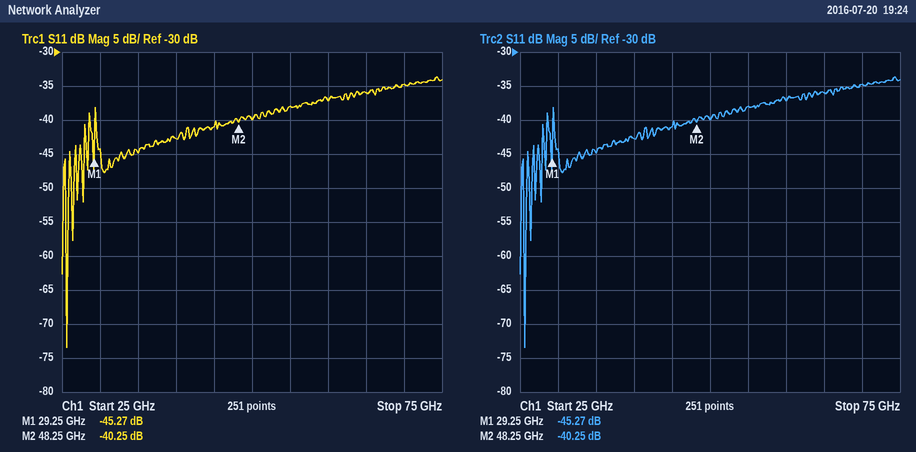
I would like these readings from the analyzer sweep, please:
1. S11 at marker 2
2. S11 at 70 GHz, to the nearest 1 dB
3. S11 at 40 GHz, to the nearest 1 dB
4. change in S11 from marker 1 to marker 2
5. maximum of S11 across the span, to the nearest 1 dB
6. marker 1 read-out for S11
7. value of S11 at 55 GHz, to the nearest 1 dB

-40.25 dB
-35 dB
-43 dB
5.02 dB
-34 dB
-45.27 dB
-38 dB
